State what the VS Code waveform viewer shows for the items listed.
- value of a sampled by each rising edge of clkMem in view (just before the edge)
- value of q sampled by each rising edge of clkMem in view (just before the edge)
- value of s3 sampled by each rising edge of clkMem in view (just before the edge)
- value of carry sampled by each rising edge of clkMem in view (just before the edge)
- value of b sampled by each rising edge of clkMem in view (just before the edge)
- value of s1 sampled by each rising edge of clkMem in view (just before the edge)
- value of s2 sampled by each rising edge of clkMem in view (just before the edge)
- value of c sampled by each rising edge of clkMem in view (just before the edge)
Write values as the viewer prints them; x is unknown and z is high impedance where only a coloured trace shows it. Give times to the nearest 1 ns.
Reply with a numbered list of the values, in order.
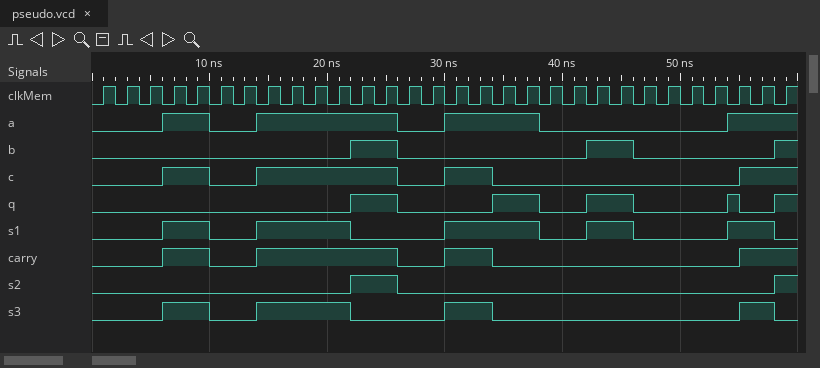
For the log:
1. 0 0 0 1 1 0 0 1 1 1 1 1 1 0 0 1 1 1 1 0 0 0 0 0 0 0 0 1 1 1
2. 0 0 0 0 0 0 0 0 0 0 0 1 1 0 0 0 0 1 1 0 0 1 1 0 0 0 0 1 0 1
3. 0 0 0 1 1 0 0 1 1 1 1 0 0 0 0 1 1 0 0 0 0 0 0 0 0 0 0 0 1 0
4. 0 0 0 1 1 0 0 1 1 1 1 1 1 0 0 1 1 0 0 0 0 0 0 0 0 0 0 0 1 1
5. 0 0 0 0 0 0 0 0 0 0 0 1 1 0 0 0 0 0 0 0 0 1 1 0 0 0 0 0 0 1
6. 0 0 0 1 1 0 0 1 1 1 1 0 0 0 0 1 1 1 1 0 0 1 1 0 0 0 0 1 1 0
7. 0 0 0 0 0 0 0 0 0 0 0 1 1 0 0 0 0 0 0 0 0 0 0 0 0 0 0 0 0 1
8. 0 0 0 1 1 0 0 1 1 1 1 1 1 0 0 1 1 0 0 0 0 0 0 0 0 0 0 0 1 1
